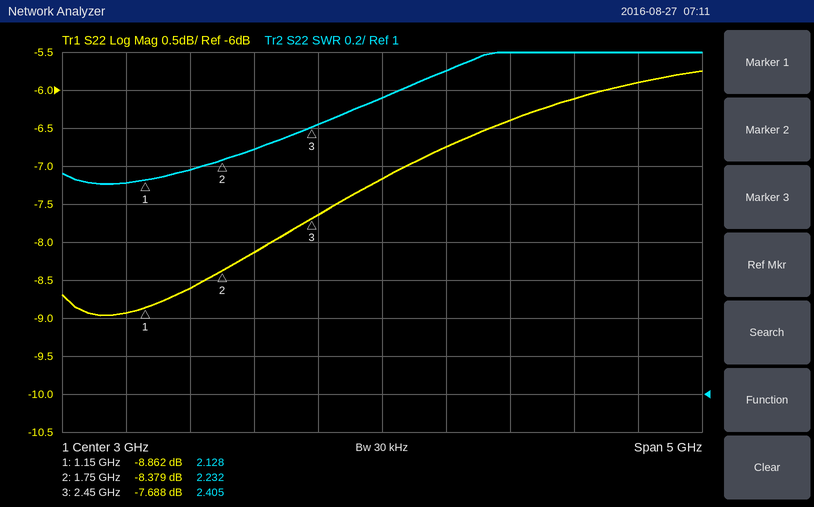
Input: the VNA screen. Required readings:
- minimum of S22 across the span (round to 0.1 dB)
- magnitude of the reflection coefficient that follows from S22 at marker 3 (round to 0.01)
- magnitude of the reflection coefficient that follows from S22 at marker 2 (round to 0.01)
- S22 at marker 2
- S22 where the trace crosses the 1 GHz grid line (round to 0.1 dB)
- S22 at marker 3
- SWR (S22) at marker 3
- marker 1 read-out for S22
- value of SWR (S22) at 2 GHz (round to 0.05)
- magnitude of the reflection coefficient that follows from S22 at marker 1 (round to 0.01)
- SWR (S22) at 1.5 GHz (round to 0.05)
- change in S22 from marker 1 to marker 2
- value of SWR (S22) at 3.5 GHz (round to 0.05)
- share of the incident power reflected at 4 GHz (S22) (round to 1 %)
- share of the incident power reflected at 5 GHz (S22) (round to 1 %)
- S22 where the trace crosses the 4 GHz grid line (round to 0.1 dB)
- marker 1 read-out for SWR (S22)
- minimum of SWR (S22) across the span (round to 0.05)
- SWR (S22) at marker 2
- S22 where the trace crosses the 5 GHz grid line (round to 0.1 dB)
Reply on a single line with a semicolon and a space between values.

-9.0 dB; 0.41; 0.38; -8.379 dB; -8.9 dB; -7.688 dB; 2.405; -8.862 dB; 2.30; 0.36; 2.20; 0.483 dB; 2.70; 23 %; 26 %; -6.4 dB; 2.128; 2.10; 2.232; -5.9 dB
